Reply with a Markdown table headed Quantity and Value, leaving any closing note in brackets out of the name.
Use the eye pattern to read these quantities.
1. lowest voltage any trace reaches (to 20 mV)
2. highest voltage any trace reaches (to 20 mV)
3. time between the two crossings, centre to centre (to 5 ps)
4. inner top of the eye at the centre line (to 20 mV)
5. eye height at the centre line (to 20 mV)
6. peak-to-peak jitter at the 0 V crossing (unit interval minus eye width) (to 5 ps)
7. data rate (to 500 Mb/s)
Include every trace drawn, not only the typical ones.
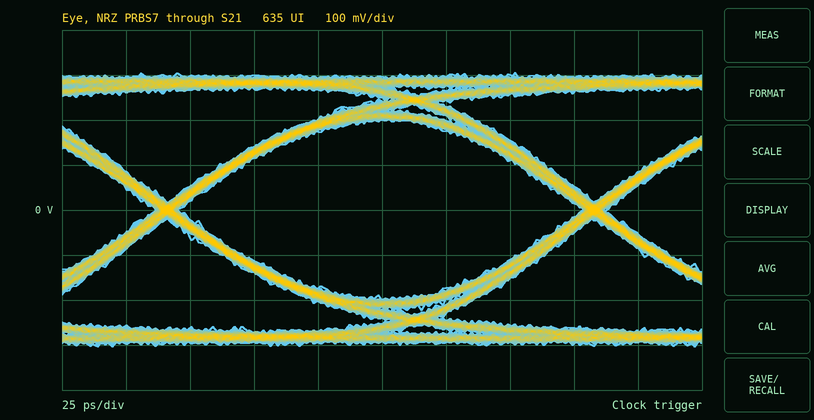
| Quantity | Value |
|---|---|
| lowest voltage any trace reaches | -300 mV |
| highest voltage any trace reaches | 300 mV |
| time between the two crossings, centre to centre | 165 ps |
| inner top of the eye at the centre line | 200 mV |
| eye height at the centre line | 400 mV |
| peak-to-peak jitter at the 0 V crossing (unit interval minus eye width) | 10 ps |
| data rate | 6.0 Gb/s |
